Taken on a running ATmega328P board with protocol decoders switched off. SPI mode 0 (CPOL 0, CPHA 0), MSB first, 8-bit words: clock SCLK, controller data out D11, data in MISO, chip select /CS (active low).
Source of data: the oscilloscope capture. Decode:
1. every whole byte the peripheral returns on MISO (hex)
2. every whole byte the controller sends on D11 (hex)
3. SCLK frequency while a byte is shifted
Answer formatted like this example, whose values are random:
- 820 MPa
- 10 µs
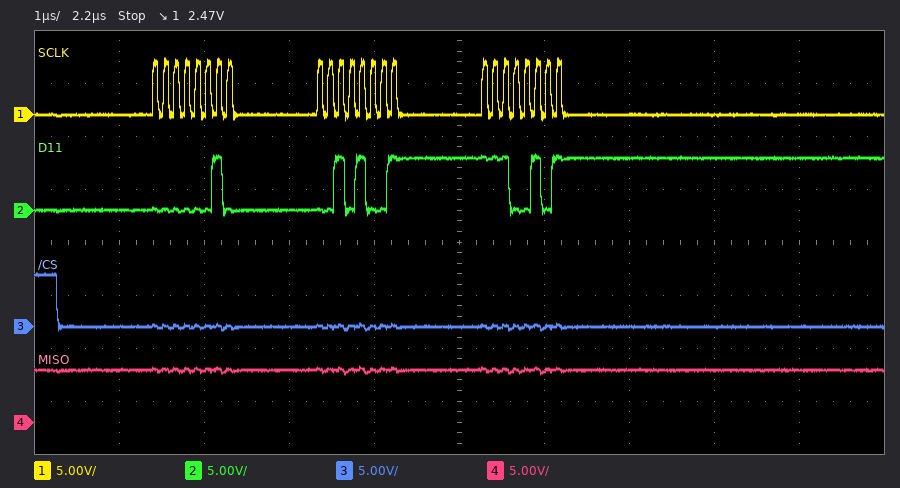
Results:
- FF FF FF
- 02 29 E5
- 8 MHz
